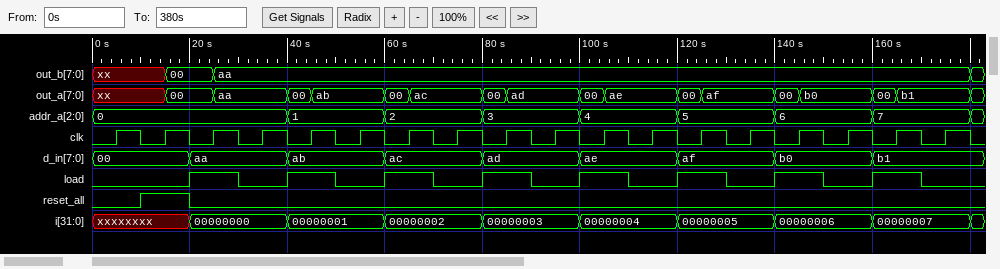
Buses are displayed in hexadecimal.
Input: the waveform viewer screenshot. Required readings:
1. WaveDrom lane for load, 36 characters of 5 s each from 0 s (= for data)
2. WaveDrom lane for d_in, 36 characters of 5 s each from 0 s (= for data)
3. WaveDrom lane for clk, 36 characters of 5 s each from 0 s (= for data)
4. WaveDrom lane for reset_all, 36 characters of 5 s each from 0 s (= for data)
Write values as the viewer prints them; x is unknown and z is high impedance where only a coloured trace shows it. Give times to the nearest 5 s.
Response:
{name: 'load', wave: '0...1.0.1.0.1.0.1.0.1.0.1.0.1.0.1.0.'}
{name: 'd_in', wave: '=...=...=...=...=...=...=...=...=...', data: '00 aa ab ac ad ae af b0 b1'}
{name: 'clk', wave: '010101010101010101010101010101010101'}
{name: 'reset_all', wave: '0.1.0...............................'}
